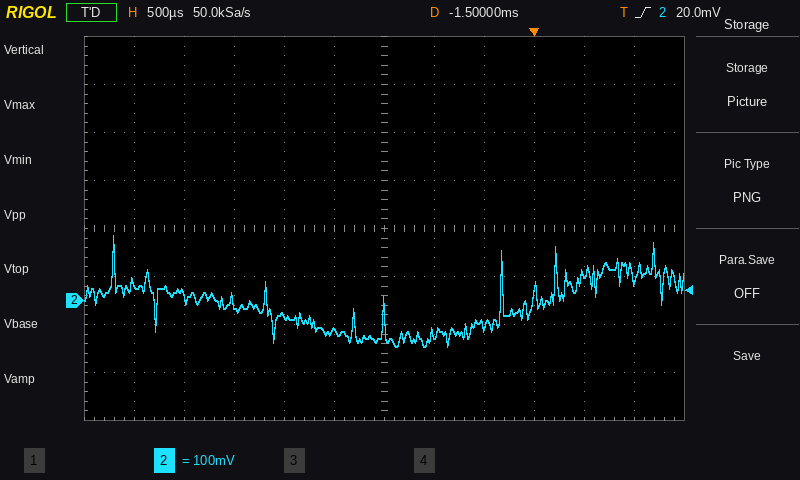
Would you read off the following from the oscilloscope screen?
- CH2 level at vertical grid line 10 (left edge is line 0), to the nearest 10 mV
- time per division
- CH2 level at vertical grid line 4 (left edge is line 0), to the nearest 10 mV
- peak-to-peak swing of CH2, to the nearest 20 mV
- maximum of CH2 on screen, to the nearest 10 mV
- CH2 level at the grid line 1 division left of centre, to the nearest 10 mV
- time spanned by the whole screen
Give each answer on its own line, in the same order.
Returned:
60 mV
500 µs
-30 mV
240 mV
140 mV
-60 mV
6 ms
